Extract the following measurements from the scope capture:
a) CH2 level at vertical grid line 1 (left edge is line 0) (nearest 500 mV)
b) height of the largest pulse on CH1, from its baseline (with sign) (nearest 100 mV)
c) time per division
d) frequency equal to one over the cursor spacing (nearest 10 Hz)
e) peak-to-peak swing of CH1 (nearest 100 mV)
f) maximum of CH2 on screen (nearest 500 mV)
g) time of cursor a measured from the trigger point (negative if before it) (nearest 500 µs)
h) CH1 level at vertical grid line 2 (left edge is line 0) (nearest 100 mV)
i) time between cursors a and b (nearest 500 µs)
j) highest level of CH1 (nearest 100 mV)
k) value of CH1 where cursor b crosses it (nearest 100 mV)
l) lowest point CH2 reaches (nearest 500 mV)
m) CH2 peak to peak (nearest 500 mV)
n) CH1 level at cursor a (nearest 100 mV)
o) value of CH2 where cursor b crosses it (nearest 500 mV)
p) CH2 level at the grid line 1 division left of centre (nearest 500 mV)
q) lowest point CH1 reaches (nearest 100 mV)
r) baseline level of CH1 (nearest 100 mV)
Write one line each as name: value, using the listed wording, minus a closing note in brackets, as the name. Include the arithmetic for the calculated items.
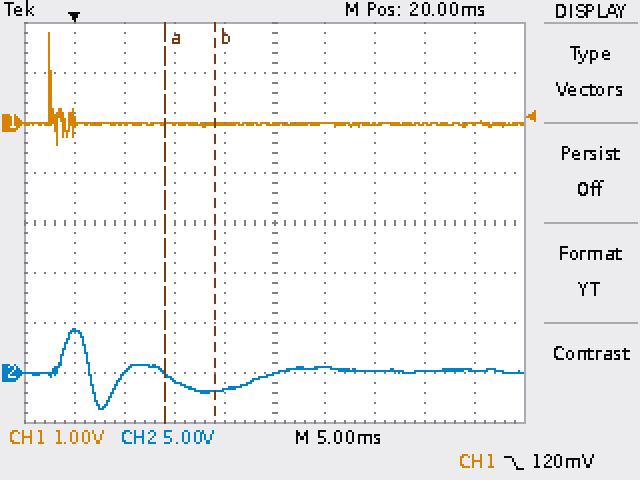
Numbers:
CH2 level at vertical grid line 1 (left edge is line 0): 4.0 V
height of the largest pulse on CH1, from its baseline (with sign): 1.8 V − (0.0 V) = +1.8 V
time per division: 5 ms
frequency equal to one over the cursor spacing: 1 / 5.0 ms ≈ 200 Hz
peak-to-peak swing of CH1: 1.8 V − (-400 mV) = 2.2 V
maximum of CH2 on screen: 4.5 V
time of cursor a measured from the trigger point (negative if before it): +9.0 ms
CH1 level at vertical grid line 2 (left edge is line 0): 0.0 V
time between cursors a and b: 5.0 ms
highest level of CH1: 1.8 V
value of CH1 where cursor b crosses it: 0.0 V
lowest point CH2 reaches: -3.5 V
CH2 peak to peak: 4.5 V − (-3.5 V) = 8.0 V
CH1 level at cursor a: 0.0 V
value of CH2 where cursor b crosses it: -2.0 V
CH2 level at the grid line 1 division left of centre: -1.5 V
lowest point CH1 reaches: -400 mV
baseline level of CH1: 0.0 V
